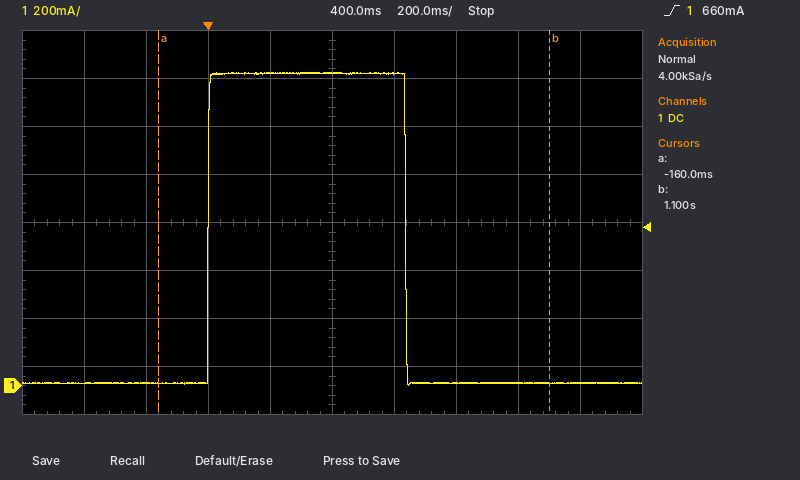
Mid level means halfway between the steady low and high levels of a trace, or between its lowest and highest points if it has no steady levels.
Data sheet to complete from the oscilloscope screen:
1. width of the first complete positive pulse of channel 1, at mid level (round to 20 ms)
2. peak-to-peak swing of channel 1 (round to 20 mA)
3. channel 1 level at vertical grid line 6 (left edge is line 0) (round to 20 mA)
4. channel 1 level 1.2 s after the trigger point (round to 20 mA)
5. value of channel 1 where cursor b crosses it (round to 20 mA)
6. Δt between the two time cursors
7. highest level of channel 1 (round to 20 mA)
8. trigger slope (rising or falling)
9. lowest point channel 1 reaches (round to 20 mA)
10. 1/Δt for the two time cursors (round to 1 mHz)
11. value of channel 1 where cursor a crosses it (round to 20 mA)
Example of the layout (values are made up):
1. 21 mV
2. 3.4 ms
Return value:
1. 640 ms
2. 1.30 A
3. 1.30 A
4. 20 mA
5. 20 mA
6. 1.26 s
7. 1.30 A
8. rising
9. 0 mA
10. 794 mHz
11. 20 mA
